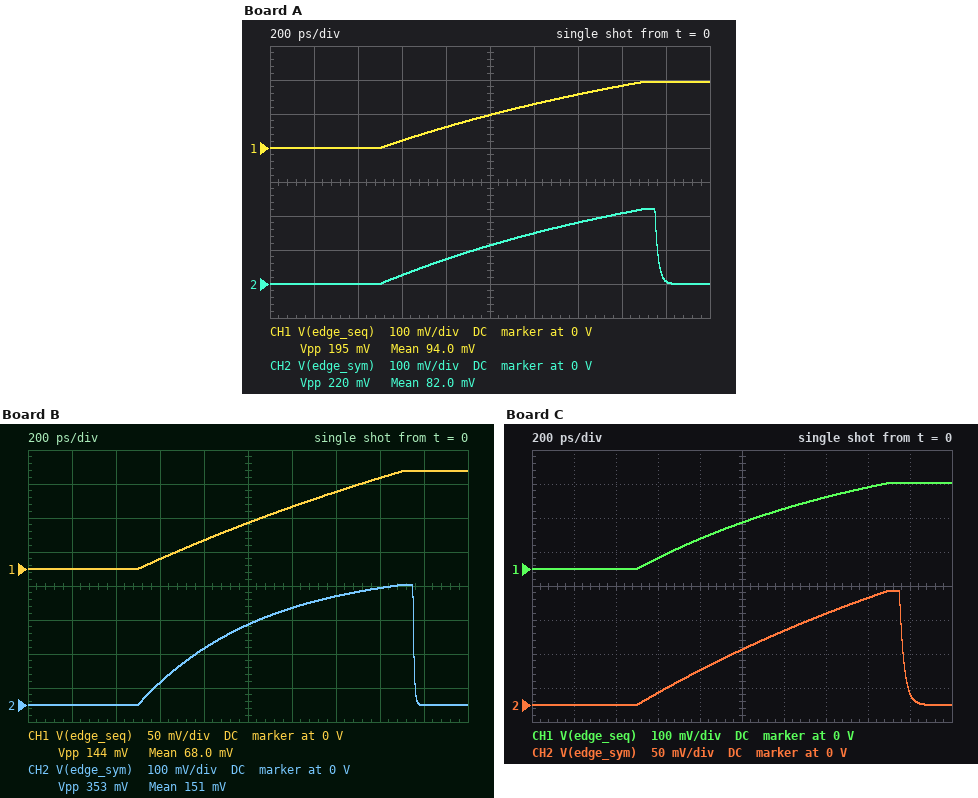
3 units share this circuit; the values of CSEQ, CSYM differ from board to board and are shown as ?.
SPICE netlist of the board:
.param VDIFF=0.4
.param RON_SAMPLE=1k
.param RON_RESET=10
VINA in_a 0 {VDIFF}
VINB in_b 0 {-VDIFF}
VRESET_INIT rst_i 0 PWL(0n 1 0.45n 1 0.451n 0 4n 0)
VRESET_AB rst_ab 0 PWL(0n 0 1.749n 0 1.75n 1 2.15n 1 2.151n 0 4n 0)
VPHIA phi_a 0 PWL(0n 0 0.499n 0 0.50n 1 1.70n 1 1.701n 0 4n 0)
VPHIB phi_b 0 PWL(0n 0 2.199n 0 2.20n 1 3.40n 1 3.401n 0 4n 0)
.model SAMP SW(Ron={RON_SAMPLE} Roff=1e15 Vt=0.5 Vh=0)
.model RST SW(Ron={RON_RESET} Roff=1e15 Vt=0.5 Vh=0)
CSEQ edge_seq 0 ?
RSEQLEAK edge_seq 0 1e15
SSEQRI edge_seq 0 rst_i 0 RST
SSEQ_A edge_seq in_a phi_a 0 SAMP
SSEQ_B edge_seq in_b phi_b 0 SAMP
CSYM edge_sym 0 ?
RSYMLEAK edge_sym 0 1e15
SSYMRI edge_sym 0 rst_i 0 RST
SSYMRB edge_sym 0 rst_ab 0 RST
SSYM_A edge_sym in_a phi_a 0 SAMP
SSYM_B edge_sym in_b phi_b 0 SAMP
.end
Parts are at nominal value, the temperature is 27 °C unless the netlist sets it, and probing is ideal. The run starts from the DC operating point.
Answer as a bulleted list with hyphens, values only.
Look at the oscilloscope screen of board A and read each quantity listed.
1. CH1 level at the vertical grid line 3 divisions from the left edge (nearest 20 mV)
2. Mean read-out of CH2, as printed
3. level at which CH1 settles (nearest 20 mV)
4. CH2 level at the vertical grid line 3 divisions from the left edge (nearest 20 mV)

- 20 mV
- 82.0 mV
- 200 mV
- 20 mV
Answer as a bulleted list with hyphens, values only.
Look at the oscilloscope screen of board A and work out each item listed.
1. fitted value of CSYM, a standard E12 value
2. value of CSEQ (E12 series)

- 1.5 pF
- 1.8 pF
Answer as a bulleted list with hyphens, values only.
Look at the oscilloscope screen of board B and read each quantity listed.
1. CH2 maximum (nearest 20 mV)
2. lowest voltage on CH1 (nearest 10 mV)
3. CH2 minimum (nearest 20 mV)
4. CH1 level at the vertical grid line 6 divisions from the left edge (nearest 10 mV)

- 360 mV
- 0 V
- 0 V
- 90 mV
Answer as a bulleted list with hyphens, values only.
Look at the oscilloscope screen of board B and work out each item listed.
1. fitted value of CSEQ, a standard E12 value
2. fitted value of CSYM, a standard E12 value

- 2.7 pF
- 560 fF
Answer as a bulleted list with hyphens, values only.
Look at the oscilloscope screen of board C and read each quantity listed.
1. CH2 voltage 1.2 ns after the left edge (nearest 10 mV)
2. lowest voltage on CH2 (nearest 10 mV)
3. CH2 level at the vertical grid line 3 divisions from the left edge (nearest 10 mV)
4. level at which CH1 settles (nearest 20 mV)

- 110 mV
- 0 V
- 20 mV
- 260 mV
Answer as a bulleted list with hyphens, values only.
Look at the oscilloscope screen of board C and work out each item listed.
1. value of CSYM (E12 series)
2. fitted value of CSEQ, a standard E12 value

- 2.2 pF
- 1.2 pF
